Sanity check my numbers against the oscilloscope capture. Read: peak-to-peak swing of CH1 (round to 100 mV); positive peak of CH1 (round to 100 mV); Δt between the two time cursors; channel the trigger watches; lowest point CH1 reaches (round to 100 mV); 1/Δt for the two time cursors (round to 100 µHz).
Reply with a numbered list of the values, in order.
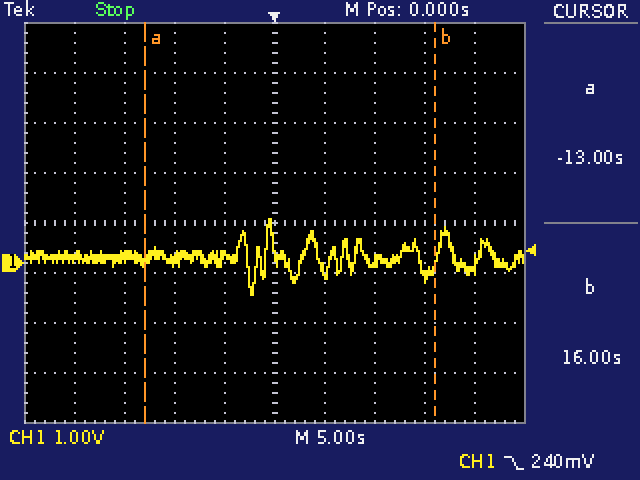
1. 1.5 V
2. 900 mV
3. 29.0 s
4. CH1
5. -600 mV
6. 34.5 mHz
